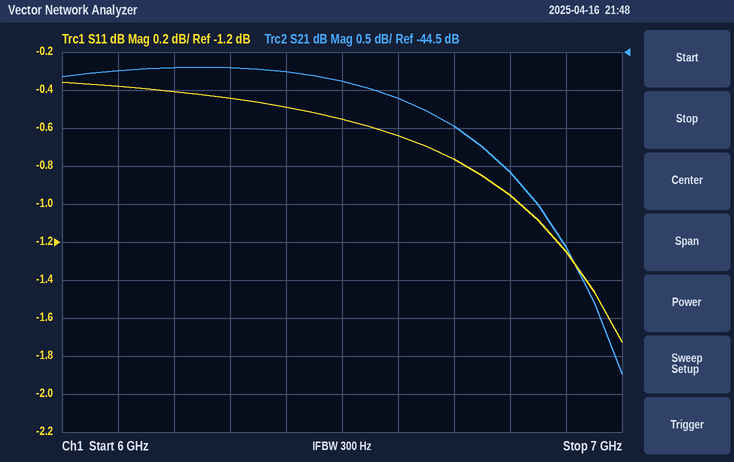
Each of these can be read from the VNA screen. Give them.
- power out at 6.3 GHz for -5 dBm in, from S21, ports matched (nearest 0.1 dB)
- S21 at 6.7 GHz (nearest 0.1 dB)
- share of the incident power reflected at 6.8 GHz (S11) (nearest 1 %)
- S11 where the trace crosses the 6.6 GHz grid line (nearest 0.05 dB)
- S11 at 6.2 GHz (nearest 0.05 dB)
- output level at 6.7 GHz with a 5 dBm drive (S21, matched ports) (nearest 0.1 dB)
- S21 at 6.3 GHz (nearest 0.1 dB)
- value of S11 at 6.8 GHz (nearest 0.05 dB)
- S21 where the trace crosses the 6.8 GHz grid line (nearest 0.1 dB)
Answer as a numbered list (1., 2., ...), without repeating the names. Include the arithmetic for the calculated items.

1. -5 dBm + (-44.7 dB) = -49.7 dBm
2. -45.5 dB
3. 10^(-0.95/10) ≈ 80 %
4. -0.65 dB
5. -0.40 dB
6. 5 dBm + (-45.5 dB) = -40.5 dBm
7. -44.7 dB
8. -0.95 dB
9. -46.1 dB
